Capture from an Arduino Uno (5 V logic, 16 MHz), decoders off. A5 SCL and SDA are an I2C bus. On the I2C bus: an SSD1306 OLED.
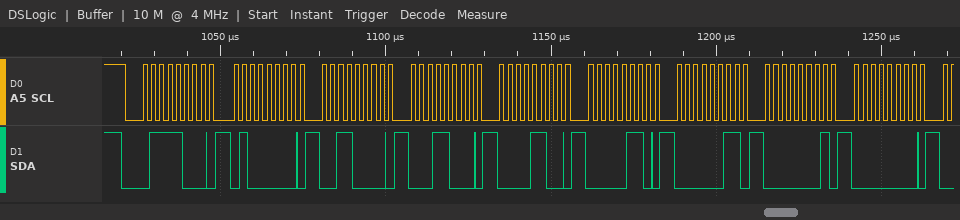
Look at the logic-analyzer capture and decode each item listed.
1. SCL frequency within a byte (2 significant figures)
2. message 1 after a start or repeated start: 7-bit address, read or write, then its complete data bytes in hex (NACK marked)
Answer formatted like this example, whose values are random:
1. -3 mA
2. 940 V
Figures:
1. 400 kHz
2. 0x3C write: 40 30 18 0C 06 03 01 00
